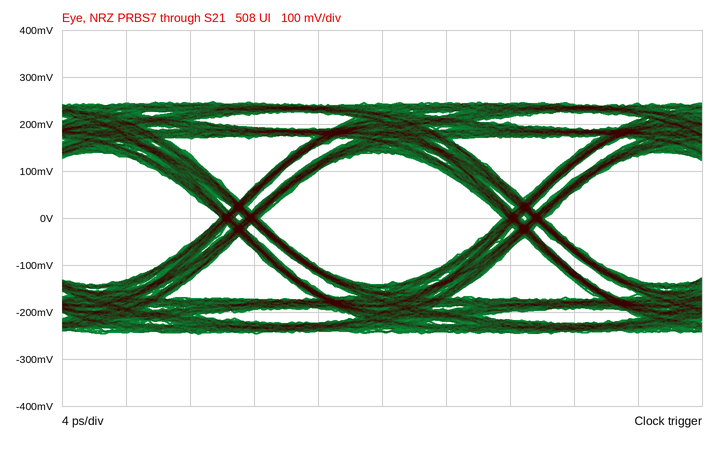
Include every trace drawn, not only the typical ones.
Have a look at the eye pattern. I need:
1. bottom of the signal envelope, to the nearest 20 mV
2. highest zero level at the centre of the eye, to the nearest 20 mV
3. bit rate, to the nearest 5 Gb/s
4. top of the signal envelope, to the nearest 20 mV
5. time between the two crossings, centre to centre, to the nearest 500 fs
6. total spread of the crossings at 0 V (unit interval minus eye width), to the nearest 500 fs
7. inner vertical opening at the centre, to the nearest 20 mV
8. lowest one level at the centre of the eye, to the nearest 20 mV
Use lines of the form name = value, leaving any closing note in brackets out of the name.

bottom of the signal envelope, to the nearest 20 mV = -240 mV
highest zero level at the centre of the eye, to the nearest 20 mV = -140 mV
bit rate, to the nearest 5 Gb/s = 55 Gb/s
top of the signal envelope, to the nearest 20 mV = 240 mV
time between the two crossings, centre to centre, to the nearest 500 fs = 18.0 ps
total spread of the crossings at 0 V (unit interval minus eye width), to the nearest 500 fs = 2.5 ps
inner vertical opening at the centre, to the nearest 20 mV = 280 mV
lowest one level at the centre of the eye, to the nearest 20 mV = 140 mV
